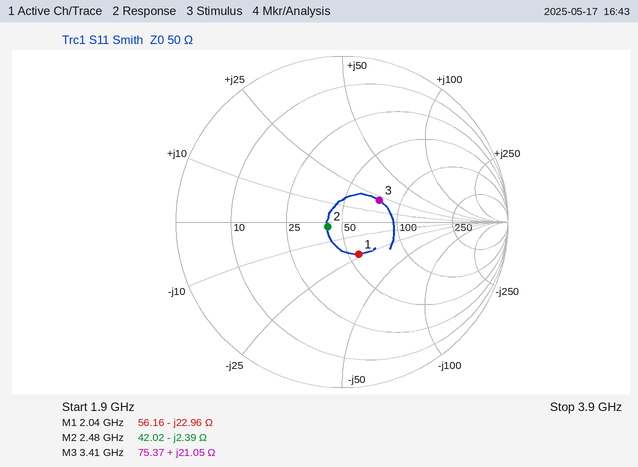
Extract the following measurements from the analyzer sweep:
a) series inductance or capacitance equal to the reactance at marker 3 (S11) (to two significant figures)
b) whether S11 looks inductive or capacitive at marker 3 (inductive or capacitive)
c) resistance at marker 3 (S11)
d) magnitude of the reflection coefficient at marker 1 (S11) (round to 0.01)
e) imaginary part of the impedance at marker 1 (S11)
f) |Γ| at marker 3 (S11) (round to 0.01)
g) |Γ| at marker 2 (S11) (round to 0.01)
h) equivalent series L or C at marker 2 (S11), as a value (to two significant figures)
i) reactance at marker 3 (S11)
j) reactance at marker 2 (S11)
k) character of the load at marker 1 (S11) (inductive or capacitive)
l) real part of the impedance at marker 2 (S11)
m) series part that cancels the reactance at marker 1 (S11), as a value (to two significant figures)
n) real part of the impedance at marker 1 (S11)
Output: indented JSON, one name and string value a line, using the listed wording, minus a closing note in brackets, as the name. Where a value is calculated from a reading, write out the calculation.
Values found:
{
  "series inductance or capacitance equal to the reactance at marker 3 (S11)": "L = 21.05 Ω/(2π × 3.41 GHz) ≈ 982 pH, so 980 pH to two significant figures",
  "whether S11 looks inductive or capacitive at marker 3": "inductive",
  "resistance at marker 3": "75.37 Ω",
  "magnitude of the reflection coefficient at marker 1 (S11)": "0.22",
  "imaginary part of the impedance at marker 1": "-22.96 Ω",
  "|Γ| at marker 3 (S11)": "0.26",
  "|Γ| at marker 2 (S11)": "0.09",
  "equivalent series L or C at marker 2 (S11), as a value": "C = 1/(2π × 2.48 GHz × 2.39 Ω) ≈ 27 pF",
  "reactance at marker 3": "+21.05 Ω",
  "reactance at marker 2": "-2.39 Ω",
  "character of the load at marker 1 (S11)": "capacitive",
  "real part of the impedance at marker 2": "42.02 Ω",
  "series part that cancels the reactance at marker 1 (S11), as a value": "L = 22.96 Ω/(2π × 2.04 GHz) ≈ 1.8 nH",
  "real part of the impedance at marker 1": "56.16 Ω"
}
